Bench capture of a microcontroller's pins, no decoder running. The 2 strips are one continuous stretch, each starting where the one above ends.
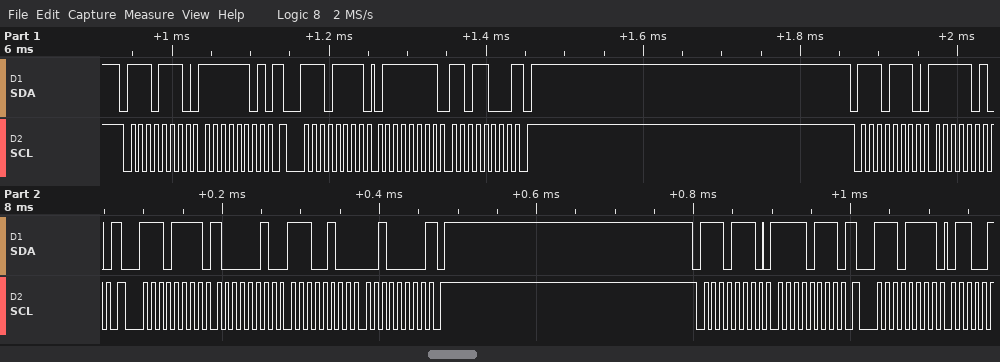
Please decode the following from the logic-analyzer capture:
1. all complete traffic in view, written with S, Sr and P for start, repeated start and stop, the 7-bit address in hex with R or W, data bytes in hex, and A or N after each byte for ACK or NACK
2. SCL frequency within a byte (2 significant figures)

S 77W A FD A Sr 77R A 7F A D8 N P S 77W A FA A Sr 77R A 82 A E4 A 20 N P S 77W A F7 A Sr 77R A
100 kHz
